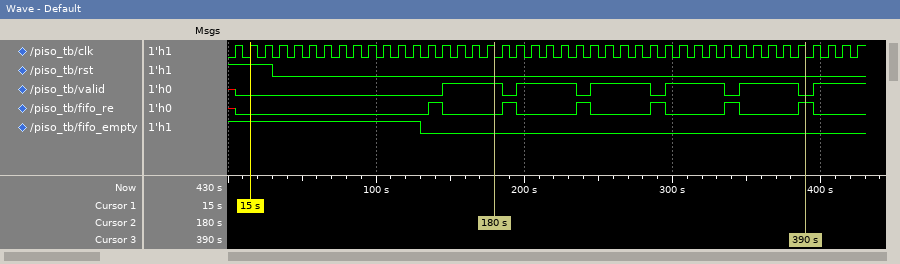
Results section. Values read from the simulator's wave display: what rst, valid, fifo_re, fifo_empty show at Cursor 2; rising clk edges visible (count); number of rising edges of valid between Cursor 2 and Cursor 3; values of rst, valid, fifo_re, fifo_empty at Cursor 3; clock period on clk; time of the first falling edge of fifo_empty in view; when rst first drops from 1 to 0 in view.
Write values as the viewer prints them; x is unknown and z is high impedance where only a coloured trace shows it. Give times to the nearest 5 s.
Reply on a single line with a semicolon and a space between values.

rst=0, valid=1, fifo_re=0, fifo_empty=0; 43; 4; rst=0, valid=0, fifo_re=1, fifo_empty=0; 10 s; 130 s; 30 s
